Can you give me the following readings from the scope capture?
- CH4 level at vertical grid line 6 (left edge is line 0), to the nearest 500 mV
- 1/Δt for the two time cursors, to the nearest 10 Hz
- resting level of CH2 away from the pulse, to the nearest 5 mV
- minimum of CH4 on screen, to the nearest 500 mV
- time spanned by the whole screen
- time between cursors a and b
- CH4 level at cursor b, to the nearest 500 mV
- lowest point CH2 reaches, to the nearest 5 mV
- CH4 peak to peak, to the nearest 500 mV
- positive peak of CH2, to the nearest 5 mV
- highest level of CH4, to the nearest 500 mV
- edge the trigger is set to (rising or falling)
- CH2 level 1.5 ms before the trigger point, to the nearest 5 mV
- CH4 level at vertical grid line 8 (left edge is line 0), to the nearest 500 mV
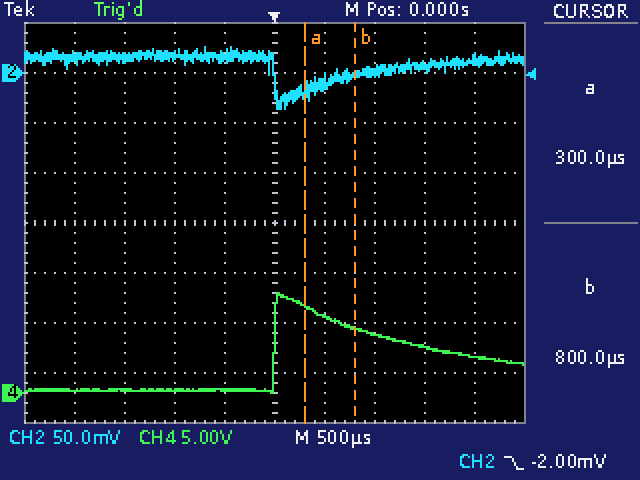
7.5 V
2.00 kHz
15 mV
0.0 V
5 ms
500 µs
6.5 V
-35 mV
10.0 V
25 mV
10.0 V
falling
15 mV
4.5 V
